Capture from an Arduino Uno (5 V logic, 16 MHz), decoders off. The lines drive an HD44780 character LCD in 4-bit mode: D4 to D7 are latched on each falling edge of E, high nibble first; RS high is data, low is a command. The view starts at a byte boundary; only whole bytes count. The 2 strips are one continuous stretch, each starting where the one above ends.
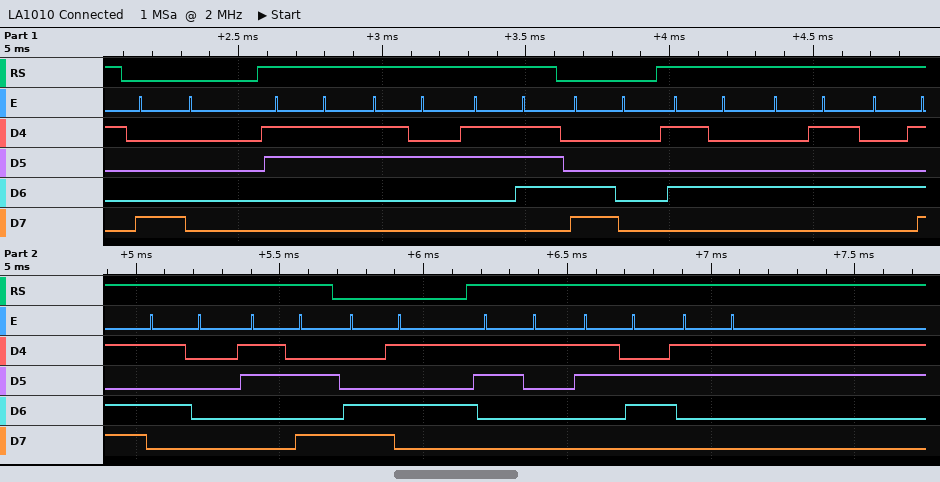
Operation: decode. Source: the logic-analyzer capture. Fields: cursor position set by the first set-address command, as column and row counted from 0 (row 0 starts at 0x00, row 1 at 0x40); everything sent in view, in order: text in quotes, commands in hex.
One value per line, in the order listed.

column 0, row 0
0x80 "327" 0xC0 "TEMP:" 0xC5 "163"
